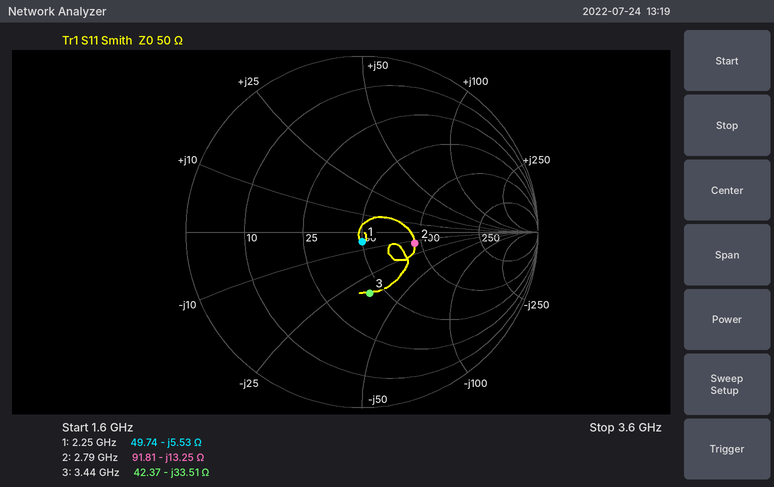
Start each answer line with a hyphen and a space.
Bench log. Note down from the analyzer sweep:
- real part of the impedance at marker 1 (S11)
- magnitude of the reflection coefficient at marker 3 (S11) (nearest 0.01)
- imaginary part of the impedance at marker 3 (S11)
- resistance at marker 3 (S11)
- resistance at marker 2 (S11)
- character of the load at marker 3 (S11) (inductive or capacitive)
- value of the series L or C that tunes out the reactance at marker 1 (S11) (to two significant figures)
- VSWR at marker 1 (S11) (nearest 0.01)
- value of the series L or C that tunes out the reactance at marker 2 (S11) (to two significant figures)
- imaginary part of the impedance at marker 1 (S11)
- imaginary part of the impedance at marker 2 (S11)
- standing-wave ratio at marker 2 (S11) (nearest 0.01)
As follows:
- 49.74 Ω
- 0.35
- -33.51 Ω
- 42.37 Ω
- 91.81 Ω
- capacitive
- 390 pH
- 1.12
- 760 pH
- -5.53 Ω
- -13.25 Ω
- 1.89
